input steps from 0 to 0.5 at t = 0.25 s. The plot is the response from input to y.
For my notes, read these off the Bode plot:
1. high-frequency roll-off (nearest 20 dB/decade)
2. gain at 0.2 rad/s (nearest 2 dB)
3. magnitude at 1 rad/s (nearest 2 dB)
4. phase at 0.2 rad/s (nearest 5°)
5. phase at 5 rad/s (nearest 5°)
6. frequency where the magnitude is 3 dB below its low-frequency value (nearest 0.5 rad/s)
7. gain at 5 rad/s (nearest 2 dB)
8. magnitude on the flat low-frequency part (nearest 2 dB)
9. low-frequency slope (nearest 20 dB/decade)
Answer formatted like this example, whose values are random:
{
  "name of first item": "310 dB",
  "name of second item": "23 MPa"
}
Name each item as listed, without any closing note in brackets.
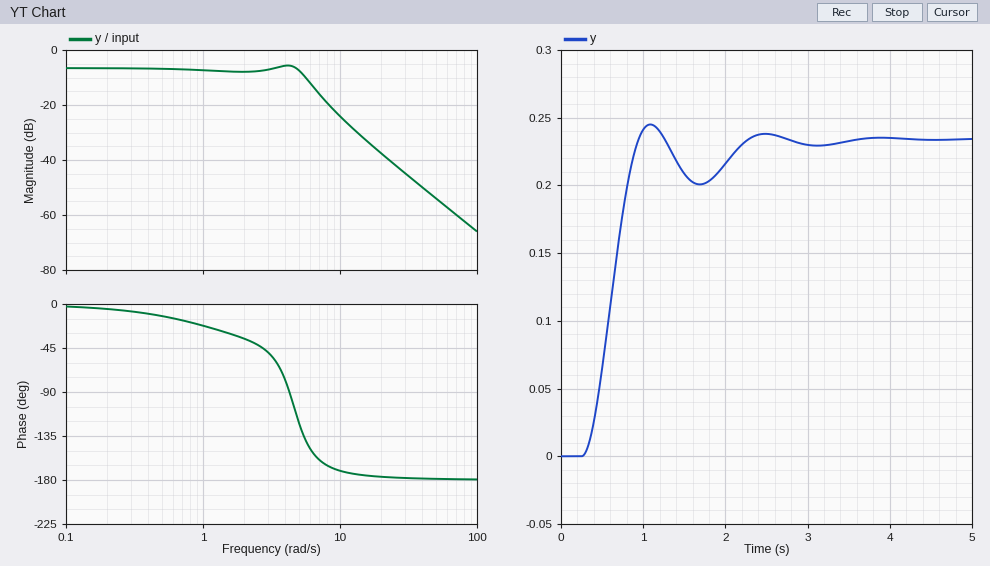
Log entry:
{
  "high-frequency roll-off": "-40 dB/decade",
  "gain at 0.2 rad/s": "-6 dB",
  "magnitude at 1 rad/s": "-8 dB",
  "phase at 0.2 rad/s": "-5°",
  "phase at 5 rad/s": "-120°",
  "frequency where the magnitude is 3 dB below its low-frequency value": "5.5 rad/s",
  "gain at 5 rad/s": "-8 dB",
  "magnitude on the flat low-frequency part": "-6 dB",
  "low-frequency slope": "0 dB/decade"
}
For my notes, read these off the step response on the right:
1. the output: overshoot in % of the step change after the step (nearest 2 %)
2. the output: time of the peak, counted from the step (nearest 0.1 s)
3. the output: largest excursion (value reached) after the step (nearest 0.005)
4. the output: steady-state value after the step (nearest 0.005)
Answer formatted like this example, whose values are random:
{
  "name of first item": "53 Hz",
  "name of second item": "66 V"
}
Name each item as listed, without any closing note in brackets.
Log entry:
{
  "the output: overshoot in % of the step change after the step": "4 %",
  "the output: time of the peak, counted from the step": "0.8 s",
  "the output: largest excursion (value reached) after the step": "0.245",
  "the output: steady-state value after the step": "0.235"
}
